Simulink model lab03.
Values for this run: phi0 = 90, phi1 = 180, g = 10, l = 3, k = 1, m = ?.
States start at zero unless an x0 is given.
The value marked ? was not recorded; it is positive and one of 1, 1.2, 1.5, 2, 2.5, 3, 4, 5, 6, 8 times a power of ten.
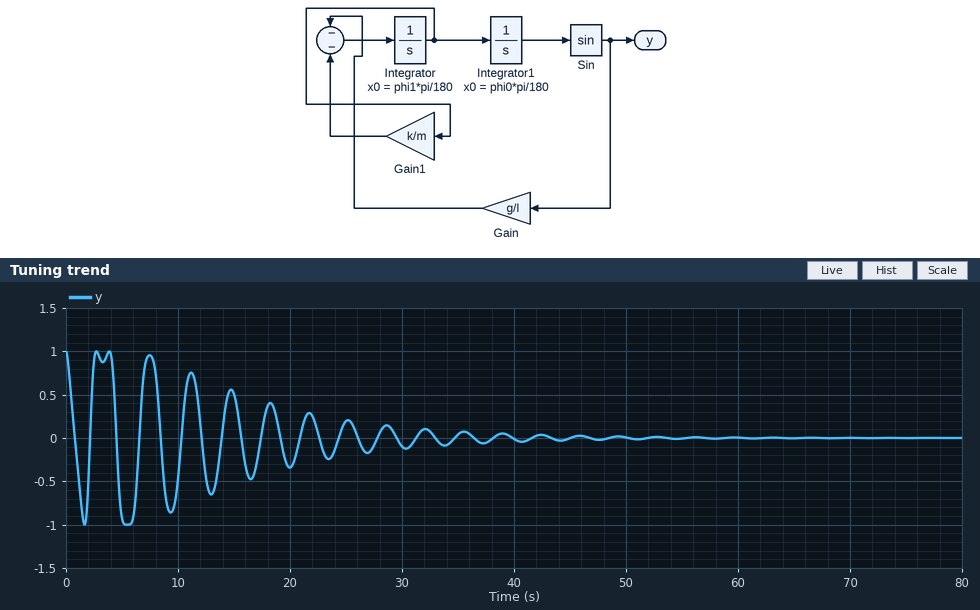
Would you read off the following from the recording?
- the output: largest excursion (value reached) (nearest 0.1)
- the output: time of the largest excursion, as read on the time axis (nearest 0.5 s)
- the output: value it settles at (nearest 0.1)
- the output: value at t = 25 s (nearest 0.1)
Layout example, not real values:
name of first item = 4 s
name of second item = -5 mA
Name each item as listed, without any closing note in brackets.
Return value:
the output: largest excursion (value reached) = -1.0
the output: time of the largest excursion, as read on the time axis = 5.5 s
the output: value it settles at = 0.0
the output: value at t = 25 s = 0.2
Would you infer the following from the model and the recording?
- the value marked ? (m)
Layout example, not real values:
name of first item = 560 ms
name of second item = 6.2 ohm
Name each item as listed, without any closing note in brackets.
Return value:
the value marked ? = 5
